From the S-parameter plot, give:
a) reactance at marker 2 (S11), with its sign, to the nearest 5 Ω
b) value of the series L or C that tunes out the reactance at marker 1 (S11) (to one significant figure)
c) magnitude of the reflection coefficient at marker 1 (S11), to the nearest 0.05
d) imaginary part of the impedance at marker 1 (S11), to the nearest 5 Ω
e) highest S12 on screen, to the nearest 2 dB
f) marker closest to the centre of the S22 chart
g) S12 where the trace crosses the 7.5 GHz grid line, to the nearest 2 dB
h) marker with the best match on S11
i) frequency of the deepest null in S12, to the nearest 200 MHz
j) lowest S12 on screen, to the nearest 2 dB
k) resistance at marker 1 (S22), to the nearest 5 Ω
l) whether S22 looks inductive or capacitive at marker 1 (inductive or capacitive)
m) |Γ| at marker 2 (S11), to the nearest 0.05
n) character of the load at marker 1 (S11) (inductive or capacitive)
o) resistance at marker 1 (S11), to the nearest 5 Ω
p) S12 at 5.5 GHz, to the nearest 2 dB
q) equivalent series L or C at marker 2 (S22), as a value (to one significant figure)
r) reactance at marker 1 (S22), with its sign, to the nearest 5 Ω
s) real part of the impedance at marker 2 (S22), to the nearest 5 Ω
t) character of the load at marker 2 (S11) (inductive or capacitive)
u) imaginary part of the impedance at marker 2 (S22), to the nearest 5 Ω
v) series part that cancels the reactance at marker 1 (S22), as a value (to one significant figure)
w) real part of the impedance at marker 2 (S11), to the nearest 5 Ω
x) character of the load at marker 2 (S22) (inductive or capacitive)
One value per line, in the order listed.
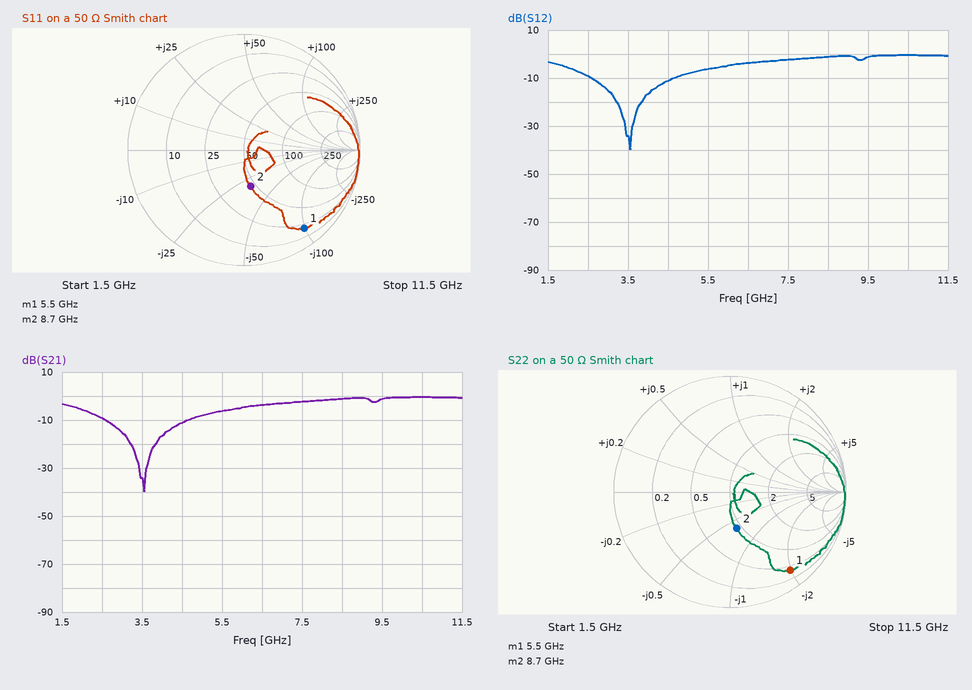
-30 Ω
3 nH
0.85
-100 Ω
0 dB
marker 2
-2 dB
marker 2
3.6 GHz
-40 dB
20 Ω
capacitive
0.30
capacitive
20 Ω
-6 dB
600 fF
-100 Ω
45 Ω
capacitive
-30 Ω
3 nH
45 Ω
capacitive
